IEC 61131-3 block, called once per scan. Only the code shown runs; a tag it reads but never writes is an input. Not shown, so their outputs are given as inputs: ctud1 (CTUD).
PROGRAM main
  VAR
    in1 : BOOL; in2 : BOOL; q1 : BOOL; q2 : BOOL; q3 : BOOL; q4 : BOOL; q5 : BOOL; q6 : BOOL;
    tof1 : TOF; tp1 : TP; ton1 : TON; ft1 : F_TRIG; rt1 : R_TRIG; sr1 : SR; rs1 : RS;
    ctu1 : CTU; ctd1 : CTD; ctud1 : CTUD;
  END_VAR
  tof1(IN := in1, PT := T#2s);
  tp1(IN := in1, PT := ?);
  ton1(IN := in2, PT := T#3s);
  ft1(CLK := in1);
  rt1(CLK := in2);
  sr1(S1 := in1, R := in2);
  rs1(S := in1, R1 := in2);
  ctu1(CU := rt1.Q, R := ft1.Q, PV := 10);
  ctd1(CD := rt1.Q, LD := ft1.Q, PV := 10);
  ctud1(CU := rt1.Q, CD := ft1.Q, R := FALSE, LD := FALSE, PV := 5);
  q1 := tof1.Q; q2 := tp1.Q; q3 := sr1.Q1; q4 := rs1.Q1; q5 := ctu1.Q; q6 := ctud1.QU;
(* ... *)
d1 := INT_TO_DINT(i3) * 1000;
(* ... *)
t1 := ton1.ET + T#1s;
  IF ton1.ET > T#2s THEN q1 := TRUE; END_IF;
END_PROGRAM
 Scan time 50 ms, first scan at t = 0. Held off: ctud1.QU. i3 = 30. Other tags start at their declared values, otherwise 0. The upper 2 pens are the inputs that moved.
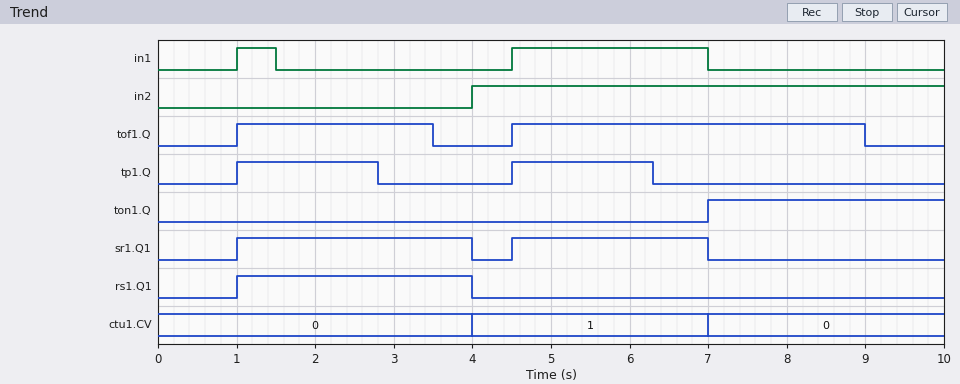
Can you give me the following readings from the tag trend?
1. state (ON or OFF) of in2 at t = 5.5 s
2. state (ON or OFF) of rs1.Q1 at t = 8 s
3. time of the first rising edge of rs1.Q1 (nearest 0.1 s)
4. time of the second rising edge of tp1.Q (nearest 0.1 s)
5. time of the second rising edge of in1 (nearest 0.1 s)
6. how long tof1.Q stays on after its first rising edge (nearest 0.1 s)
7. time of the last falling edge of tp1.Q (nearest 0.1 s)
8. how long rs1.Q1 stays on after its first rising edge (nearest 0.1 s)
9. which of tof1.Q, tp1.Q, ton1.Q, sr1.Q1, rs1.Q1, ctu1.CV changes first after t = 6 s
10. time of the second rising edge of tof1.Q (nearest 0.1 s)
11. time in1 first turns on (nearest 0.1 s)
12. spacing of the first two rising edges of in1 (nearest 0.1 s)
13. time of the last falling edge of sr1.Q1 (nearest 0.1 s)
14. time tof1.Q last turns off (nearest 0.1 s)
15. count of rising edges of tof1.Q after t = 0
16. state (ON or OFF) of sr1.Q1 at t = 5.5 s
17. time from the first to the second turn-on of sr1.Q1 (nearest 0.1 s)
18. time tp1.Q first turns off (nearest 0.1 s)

ON
OFF
1.0 s
4.5 s
4.5 s
2.5 s
6.3 s
3.0 s
tp1.Q
4.5 s
1.0 s
3.5 s
7.0 s
9.0 s
2
ON
3.5 s
2.8 s
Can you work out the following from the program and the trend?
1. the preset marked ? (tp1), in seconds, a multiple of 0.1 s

1.8 s
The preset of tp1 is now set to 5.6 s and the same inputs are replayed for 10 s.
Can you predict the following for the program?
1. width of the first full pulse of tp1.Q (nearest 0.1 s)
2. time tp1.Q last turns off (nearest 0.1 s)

5.6 s
6.6 s
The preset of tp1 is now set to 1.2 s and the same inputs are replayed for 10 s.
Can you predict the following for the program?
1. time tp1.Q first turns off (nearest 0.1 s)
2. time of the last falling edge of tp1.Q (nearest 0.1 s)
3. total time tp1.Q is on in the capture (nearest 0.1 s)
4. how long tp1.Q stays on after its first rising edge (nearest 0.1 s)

2.2 s
5.7 s
2.4 s
1.2 s
